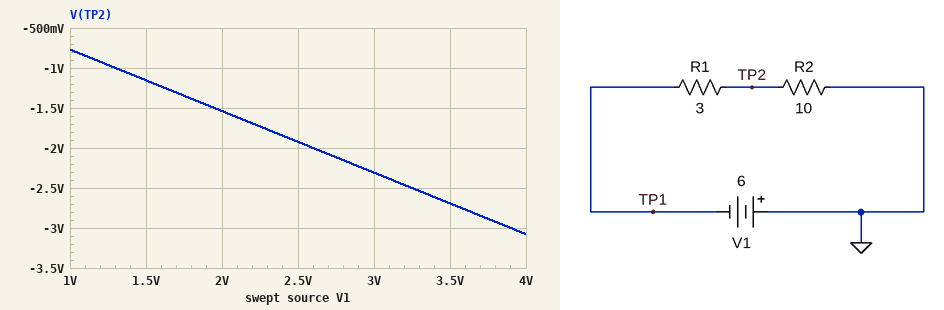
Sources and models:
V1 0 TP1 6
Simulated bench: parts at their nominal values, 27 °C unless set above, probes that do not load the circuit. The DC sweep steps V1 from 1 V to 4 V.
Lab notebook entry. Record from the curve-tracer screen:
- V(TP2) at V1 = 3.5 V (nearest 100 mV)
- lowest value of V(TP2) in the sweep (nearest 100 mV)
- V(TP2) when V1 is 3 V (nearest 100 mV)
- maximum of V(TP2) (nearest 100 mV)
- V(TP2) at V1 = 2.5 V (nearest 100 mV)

-2.7 V
-3.1 V
-2.3 V
-800 mV
-1.9 V
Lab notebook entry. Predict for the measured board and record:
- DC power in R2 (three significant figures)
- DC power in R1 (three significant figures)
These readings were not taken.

2.13 W
639 mW
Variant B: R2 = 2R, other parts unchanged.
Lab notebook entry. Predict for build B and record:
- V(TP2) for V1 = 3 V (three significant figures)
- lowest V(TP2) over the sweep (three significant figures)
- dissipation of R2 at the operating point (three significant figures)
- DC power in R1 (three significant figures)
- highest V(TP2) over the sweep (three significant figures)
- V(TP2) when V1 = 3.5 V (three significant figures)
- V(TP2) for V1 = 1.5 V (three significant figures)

-1.20 V
-1.60 V
2.88 W
4.32 W
-400 mV
-1.40 V
-600 mV
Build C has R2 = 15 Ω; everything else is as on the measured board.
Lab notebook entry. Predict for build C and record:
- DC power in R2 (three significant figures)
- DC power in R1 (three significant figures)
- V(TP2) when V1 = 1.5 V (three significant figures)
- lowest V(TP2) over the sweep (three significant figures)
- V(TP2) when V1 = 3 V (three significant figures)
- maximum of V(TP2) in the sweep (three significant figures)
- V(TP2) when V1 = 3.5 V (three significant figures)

1.67 W
333 mW
-1.25 V
-3.33 V
-2.50 V
-833 mV
-2.92 V
